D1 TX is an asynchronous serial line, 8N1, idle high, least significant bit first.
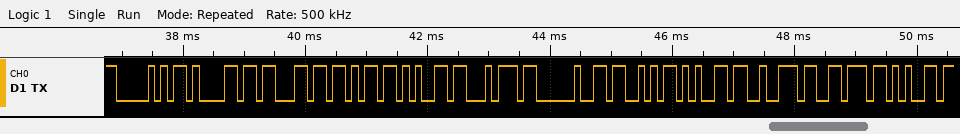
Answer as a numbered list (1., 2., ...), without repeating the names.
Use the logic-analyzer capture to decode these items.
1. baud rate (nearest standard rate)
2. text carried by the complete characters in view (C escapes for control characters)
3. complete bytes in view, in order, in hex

1. 9600 baud
2. "Packet Serve"
3. 0x50 0x61 0x63 0x6B 0x65 0x74 0x20 0x53 0x65 0x72 0x76 0x65
